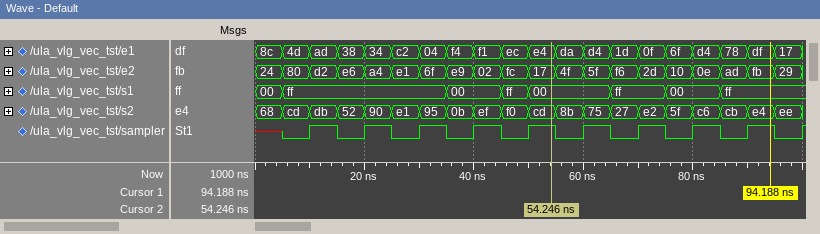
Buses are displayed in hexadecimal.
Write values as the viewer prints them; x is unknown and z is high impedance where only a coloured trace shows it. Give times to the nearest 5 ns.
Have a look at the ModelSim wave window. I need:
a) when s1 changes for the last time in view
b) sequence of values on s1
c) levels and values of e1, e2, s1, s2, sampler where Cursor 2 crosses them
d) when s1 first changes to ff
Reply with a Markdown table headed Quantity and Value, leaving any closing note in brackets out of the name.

| Quantity | Value |
|---|---|
| when s1 changes for the last time in view | 85 ns |
| sequence of values on s1 | 00, ff, 00, ff, 00, ff, 00, ff |
| levels and values of e1, e2, s1, s2, sampler where Cursor 2 crosses them | e1=e4, e2=17, s1=00, s2=cd, sampler=1 |
| when s1 first changes to ff | 5 ns |
